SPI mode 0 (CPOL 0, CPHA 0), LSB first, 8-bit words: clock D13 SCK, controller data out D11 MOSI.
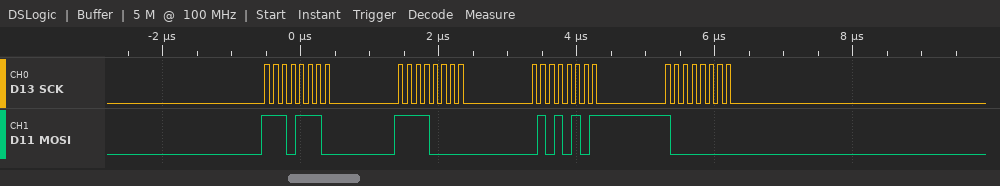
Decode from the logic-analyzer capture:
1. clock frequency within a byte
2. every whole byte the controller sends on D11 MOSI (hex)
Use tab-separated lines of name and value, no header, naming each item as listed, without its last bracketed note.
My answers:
clock frequency within a byte	8 MHz
every whole byte the controller sends on D11 MOSI	77 0F AA 01
